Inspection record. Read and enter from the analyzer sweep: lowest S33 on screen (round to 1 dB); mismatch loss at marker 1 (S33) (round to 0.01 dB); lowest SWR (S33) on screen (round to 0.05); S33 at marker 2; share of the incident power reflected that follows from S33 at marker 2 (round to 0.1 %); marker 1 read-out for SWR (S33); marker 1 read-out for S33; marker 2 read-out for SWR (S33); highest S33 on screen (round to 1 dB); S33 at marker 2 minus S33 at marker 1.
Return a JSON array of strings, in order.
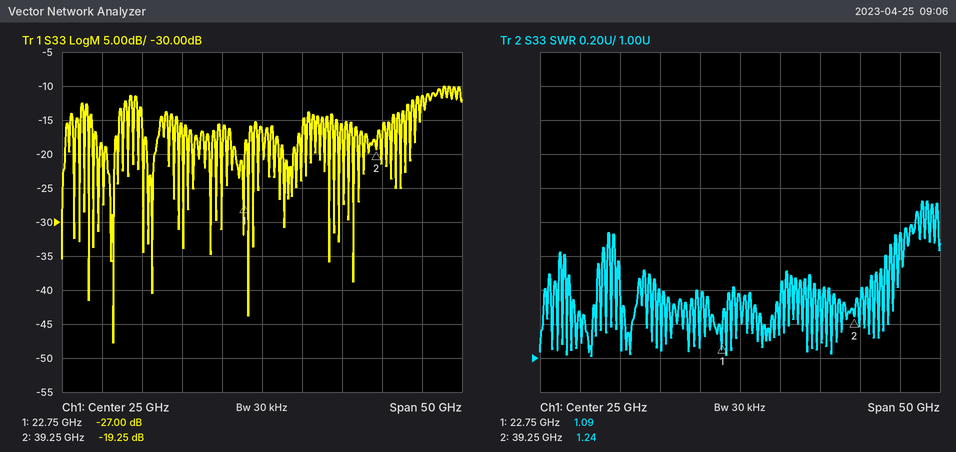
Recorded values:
["-48 dB", "0.01 dB", "1.00", "-19.25 dB", "1.2 %", "1.09", "-27.00 dB", "1.24", "-10 dB", "7.75 dB"]
